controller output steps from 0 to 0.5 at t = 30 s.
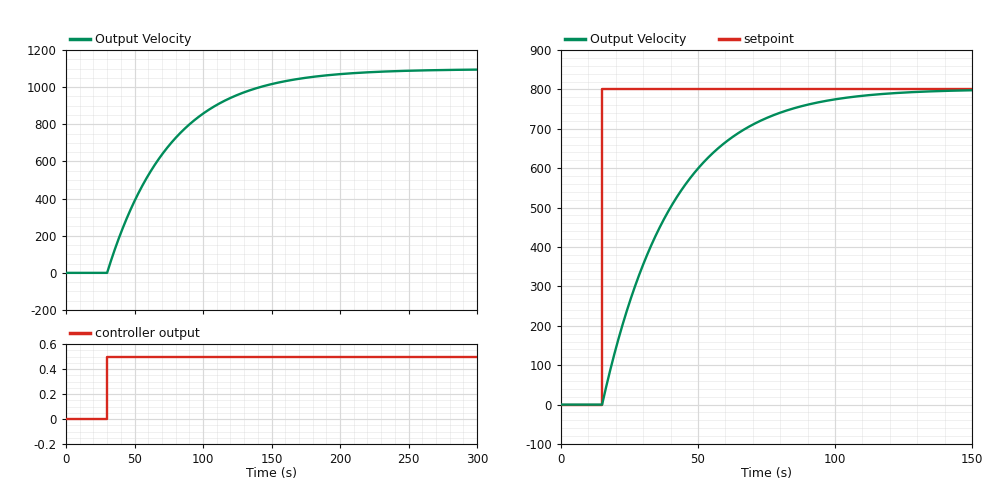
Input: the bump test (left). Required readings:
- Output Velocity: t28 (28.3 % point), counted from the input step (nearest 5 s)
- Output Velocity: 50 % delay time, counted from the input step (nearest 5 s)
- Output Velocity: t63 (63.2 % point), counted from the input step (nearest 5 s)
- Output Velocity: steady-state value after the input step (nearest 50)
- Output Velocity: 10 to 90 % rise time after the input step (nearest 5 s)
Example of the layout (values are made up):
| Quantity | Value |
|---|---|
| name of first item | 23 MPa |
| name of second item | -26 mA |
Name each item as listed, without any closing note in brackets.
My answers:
| Quantity | Value |
|---|---|
| Output Velocity: t28 (28.3 % point), counted from the input step | 15 s |
| Output Velocity: 50 % delay time, counted from the input step | 30 s |
| Output Velocity: t63 (63.2 % point), counted from the input step | 45 s |
| Output Velocity: steady-state value after the input step | 1100 |
| Output Velocity: 10 to 90 % rise time after the input step | 100 s |
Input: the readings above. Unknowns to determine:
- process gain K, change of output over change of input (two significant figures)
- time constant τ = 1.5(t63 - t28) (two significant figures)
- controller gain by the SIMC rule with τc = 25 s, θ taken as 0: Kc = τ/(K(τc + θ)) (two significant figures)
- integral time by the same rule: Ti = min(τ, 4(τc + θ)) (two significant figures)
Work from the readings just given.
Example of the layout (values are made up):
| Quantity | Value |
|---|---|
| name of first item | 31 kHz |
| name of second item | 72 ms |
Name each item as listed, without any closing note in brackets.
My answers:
| Quantity | Value |
|---|---|
| process gain K, change of output over change of input | 2200 |
| time constant τ = 1.5(t63 - t28) | 45 s |
| controller gain by the SIMC rule with τc = 25 s, θ taken as 0: Kc = τ/(K(τc + θ)) | 0.00082 |
| integral time by the same rule: Ti = min(τ, 4(τc + θ)) | 45 s |
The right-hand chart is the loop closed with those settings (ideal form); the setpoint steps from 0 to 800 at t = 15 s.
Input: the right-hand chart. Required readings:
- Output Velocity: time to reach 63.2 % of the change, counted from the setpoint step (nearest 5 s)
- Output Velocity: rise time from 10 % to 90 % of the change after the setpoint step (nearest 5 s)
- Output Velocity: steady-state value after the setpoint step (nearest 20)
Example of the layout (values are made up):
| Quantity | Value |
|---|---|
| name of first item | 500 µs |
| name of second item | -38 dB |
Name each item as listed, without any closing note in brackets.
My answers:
| Quantity | Value |
|---|---|
| Output Velocity: time to reach 63.2 % of the change, counted from the setpoint step | 25 s |
| Output Velocity: rise time from 10 % to 90 % of the change after the setpoint step | 55 s |
| Output Velocity: steady-state value after the setpoint step | 800 |
